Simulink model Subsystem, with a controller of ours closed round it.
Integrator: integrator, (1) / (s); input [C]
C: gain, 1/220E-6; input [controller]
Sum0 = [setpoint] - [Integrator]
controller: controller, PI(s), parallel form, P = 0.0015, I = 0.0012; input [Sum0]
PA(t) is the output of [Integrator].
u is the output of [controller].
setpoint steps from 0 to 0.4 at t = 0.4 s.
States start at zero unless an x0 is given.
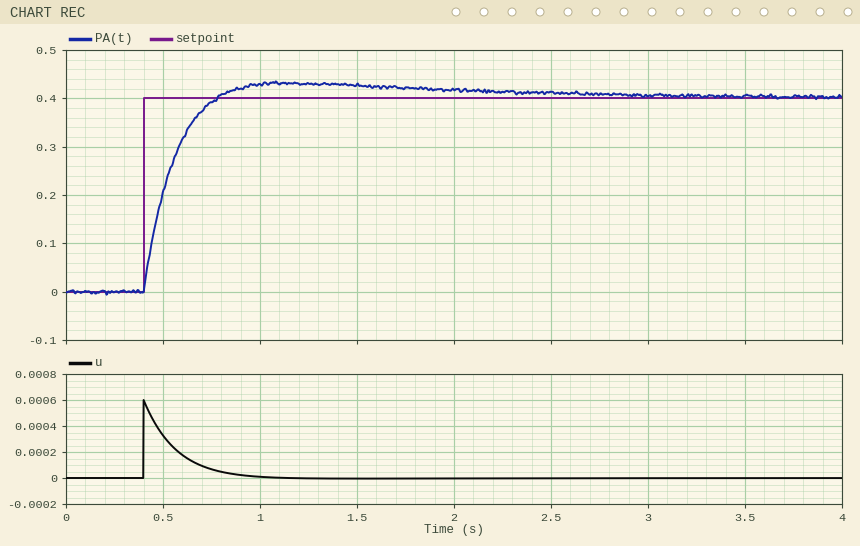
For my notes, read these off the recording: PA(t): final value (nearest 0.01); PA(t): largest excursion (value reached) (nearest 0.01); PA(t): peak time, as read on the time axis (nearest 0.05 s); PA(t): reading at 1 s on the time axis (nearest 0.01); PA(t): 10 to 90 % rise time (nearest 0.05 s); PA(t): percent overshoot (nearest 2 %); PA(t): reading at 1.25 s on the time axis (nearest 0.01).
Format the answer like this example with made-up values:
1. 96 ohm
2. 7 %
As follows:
1. 0.40
2. 0.43
3. 1.15 s
4. 0.43
5. 0.25 s
6. 8 %
7. 0.43
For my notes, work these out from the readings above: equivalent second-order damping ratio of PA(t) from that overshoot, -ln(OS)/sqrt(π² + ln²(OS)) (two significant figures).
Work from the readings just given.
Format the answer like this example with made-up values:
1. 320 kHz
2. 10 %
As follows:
1. 0.63
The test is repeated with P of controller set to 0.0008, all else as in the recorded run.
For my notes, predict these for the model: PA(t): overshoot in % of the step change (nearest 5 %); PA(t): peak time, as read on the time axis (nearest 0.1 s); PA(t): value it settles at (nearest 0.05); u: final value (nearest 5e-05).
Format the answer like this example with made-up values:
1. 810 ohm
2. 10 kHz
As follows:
1. 20 %
2. 1.3 s
3. 0.40
4. 0.00000
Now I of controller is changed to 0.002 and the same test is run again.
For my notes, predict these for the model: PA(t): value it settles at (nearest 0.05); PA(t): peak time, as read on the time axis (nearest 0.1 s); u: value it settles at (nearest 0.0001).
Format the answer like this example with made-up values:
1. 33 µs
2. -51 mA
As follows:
1. 0.40
2. 1.0 s
3. 0.0000
